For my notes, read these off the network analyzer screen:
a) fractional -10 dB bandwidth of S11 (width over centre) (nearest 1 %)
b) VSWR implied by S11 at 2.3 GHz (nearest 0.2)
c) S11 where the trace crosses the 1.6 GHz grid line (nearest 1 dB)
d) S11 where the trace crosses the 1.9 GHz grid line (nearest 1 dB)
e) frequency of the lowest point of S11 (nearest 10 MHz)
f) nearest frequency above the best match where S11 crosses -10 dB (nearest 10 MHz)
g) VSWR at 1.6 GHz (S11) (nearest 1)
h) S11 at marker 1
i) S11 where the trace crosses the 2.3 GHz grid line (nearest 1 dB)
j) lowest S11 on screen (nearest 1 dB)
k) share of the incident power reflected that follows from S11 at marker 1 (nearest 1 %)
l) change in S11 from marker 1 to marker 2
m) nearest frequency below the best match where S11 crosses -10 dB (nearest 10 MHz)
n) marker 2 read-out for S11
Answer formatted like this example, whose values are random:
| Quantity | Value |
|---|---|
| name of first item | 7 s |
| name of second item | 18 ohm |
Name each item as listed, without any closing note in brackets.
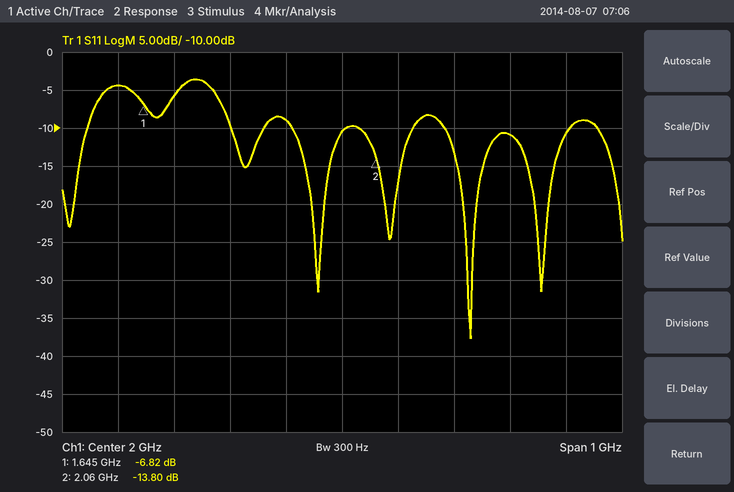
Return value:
| Quantity | Value |
|---|---|
| fractional -10 dB bandwidth of S11 (width over centre) | 10 % |
| VSWR implied by S11 at 2.3 GHz | 1.8 |
| S11 where the trace crosses the 1.6 GHz grid line | -4 dB |
| S11 where the trace crosses the 1.9 GHz grid line | -9 dB |
| frequency of the lowest point of S11 | 2.23 GHz |
| nearest frequency above the best match where S11 crosses -10 dB | 2.41 GHz |
| VSWR at 1.6 GHz (S11) | 4 |
| S11 at marker 1 | -6.82 dB |
| S11 where the trace crosses the 2.3 GHz grid line | -11 dB |
| lowest S11 on screen | -38 dB |
| share of the incident power reflected that follows from S11 at marker 1 | 21 % |
| change in S11 from marker 1 to marker 2 | -6.98 dB |
| nearest frequency below the best match where S11 crosses -10 dB | 2.18 GHz |
| marker 2 read-out for S11 | -13.80 dB |
